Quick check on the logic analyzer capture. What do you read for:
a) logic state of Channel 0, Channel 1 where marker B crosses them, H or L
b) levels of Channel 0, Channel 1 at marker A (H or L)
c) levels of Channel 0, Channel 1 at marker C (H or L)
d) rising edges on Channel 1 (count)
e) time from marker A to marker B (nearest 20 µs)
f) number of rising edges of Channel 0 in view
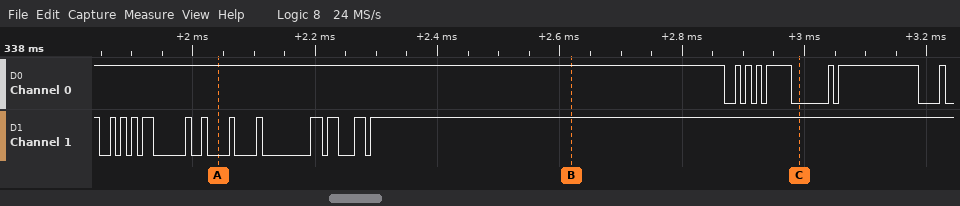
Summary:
Channel 0=H, Channel 1=H
Channel 0=H, Channel 1=L
Channel 0=L, Channel 1=H
12
580 µs
7
